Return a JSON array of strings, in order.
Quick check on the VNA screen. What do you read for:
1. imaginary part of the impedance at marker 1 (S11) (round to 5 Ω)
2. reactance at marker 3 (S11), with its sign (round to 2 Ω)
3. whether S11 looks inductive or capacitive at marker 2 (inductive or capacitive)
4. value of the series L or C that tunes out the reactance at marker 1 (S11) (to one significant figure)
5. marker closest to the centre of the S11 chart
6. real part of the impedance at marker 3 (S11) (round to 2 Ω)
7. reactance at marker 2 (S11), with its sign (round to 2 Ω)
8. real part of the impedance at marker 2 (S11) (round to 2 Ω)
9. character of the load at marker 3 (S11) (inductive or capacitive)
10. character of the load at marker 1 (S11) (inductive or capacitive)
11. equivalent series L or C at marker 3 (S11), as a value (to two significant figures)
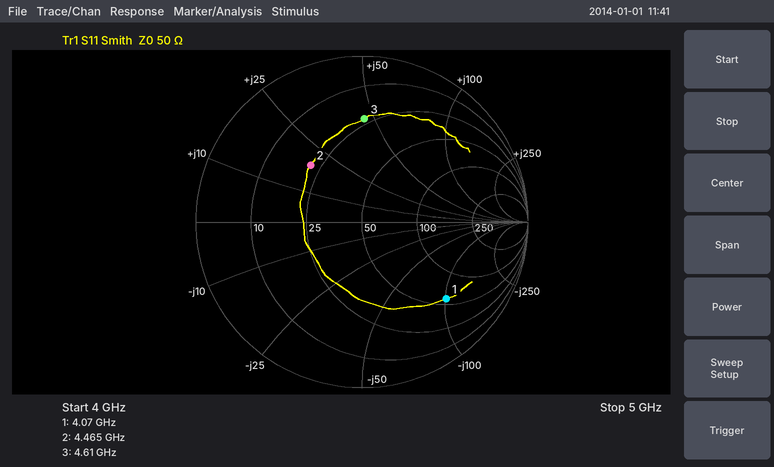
["-100 Ω", "+46 Ω", "inductive", "4 nH", "marker 2", "22 Ω", "+18 Ω", "22 Ω", "inductive", "capacitive", "1.6 nH"]
